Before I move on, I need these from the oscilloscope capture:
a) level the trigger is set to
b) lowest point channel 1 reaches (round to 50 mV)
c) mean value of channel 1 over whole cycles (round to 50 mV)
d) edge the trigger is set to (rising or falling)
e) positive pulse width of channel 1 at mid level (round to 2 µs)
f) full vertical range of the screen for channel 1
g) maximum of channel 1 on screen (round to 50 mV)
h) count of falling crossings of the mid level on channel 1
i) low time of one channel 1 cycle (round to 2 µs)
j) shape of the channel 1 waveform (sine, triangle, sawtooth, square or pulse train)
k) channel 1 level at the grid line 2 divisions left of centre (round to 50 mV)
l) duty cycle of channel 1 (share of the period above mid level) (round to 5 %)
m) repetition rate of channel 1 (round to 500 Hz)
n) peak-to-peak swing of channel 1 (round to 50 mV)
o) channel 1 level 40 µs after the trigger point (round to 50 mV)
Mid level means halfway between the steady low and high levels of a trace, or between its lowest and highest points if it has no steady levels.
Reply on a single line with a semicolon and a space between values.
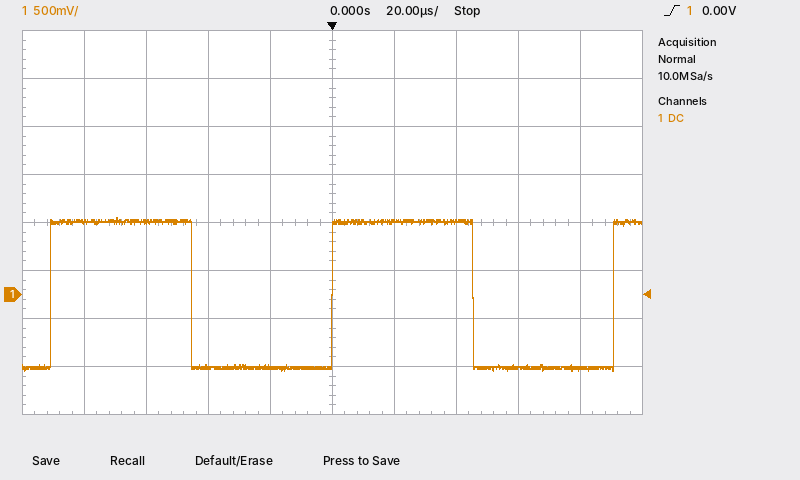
0.00 V; -800 mV; 0 mV; rising; 46 µs; 4 V; 800 mV; 2; 46 µs; square; -750 mV; 50 %; 11.0 kHz; 1.60 V; 750 mV
